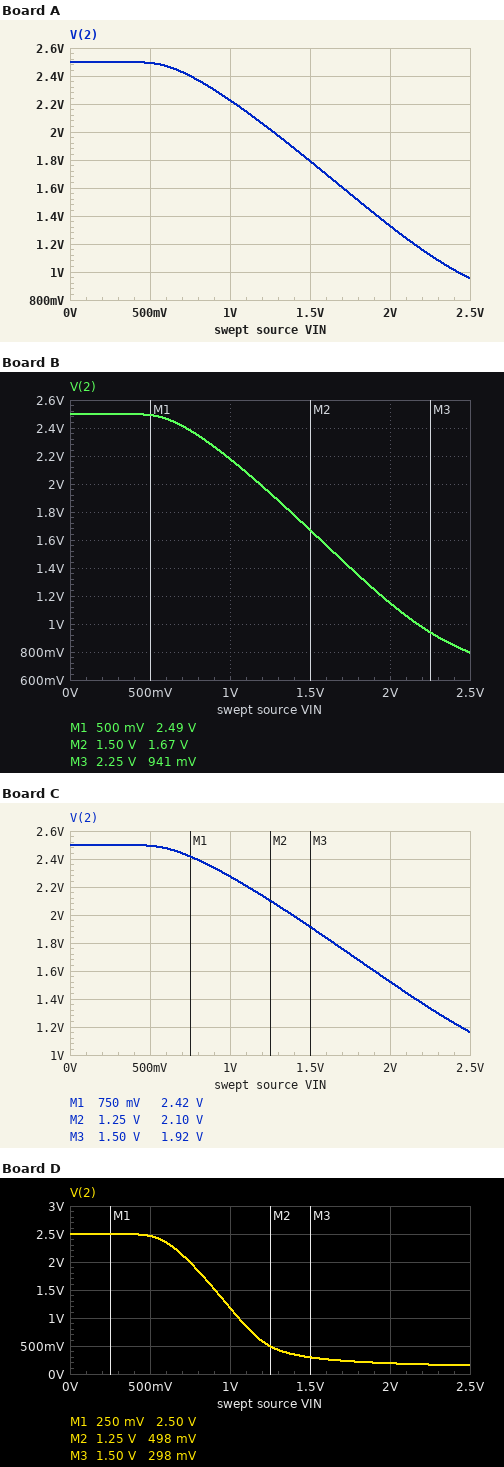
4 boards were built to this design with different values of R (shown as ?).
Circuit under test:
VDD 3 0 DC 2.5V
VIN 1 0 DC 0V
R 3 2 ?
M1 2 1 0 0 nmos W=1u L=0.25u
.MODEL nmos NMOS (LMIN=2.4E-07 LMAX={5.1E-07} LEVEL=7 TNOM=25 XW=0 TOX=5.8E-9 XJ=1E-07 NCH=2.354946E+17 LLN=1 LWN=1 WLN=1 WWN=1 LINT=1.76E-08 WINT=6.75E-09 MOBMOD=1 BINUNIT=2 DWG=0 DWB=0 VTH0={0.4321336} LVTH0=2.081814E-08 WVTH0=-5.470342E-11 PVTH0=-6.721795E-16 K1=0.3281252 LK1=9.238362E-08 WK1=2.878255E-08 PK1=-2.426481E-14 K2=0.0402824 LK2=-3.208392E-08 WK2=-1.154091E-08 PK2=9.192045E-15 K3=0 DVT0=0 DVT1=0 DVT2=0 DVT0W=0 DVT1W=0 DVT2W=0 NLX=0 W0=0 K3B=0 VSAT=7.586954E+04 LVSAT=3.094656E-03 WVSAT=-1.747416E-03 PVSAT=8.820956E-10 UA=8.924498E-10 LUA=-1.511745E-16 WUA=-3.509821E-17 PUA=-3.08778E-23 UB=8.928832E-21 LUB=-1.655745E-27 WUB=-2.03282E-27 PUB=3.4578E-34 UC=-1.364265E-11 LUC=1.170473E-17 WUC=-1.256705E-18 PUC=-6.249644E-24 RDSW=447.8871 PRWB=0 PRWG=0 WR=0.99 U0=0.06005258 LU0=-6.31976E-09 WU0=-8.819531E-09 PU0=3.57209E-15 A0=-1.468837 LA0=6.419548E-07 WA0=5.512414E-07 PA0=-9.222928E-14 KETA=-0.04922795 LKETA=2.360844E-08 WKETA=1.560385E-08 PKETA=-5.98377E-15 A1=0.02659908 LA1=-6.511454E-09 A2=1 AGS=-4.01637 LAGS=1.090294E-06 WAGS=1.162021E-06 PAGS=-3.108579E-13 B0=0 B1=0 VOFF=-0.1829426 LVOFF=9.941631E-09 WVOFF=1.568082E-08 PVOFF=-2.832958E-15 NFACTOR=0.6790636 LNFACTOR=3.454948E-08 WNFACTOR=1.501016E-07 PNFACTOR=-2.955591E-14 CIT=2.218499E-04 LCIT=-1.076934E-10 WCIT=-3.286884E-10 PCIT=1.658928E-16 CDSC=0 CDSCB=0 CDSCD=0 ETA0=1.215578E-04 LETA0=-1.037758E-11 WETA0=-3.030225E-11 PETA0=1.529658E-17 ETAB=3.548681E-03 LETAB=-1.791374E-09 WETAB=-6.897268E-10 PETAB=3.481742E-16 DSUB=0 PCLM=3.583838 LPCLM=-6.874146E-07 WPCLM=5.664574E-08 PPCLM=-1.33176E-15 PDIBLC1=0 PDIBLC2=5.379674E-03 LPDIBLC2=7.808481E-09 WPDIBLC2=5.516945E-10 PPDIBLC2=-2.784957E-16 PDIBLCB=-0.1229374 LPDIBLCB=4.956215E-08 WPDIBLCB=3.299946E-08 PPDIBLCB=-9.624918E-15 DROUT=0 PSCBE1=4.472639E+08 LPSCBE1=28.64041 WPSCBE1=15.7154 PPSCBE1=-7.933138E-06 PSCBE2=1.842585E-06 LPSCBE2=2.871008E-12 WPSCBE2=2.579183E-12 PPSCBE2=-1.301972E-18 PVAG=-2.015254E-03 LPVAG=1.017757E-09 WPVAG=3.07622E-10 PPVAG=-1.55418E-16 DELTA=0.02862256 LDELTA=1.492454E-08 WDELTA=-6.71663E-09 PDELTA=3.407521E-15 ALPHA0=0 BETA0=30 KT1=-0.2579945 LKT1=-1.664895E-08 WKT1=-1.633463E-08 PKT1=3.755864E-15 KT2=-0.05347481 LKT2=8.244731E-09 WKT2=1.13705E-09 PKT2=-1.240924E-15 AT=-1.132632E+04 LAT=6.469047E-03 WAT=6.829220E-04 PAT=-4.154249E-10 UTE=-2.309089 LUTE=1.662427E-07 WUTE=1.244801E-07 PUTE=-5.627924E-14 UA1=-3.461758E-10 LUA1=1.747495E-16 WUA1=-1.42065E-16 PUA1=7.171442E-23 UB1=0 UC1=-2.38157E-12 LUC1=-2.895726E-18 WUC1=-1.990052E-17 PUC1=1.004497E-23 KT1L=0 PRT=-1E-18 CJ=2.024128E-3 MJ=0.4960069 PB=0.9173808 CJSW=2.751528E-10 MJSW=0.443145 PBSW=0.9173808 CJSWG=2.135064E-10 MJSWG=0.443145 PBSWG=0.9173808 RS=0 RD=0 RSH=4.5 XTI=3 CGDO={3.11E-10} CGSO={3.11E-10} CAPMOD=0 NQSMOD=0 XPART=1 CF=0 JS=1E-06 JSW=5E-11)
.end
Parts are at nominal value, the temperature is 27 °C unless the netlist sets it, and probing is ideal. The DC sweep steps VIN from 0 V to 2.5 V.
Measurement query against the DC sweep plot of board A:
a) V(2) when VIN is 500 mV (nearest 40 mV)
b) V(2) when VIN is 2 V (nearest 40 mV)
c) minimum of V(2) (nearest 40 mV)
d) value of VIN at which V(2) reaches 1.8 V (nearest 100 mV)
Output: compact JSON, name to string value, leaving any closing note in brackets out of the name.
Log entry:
{"V(2) when VIN is 500 mV": "2.48 V", "V(2) when VIN is 2 V": "1.32 V", "minimum of V(2)": "960 mV", "value of VIN at which V(2) reaches 1.8 V": "1.5 V"}
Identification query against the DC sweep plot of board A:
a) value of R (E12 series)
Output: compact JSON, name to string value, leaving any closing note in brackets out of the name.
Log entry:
{"value of R": "3.3 kΩ"}
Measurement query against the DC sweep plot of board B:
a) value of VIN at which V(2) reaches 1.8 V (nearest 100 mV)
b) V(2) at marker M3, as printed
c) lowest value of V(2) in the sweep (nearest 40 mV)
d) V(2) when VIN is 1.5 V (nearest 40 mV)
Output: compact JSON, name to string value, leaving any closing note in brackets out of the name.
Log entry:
{"value of VIN at which V(2) reaches 1.8 V": "1.4 V", "V(2) at marker M3, as printed": "941 mV", "lowest value of V(2) in the sweep": "800 mV", "V(2) when VIN is 1.5 V": "1.68 V"}
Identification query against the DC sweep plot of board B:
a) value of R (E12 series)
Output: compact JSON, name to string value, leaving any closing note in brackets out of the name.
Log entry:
{"value of R": "3.9 kΩ"}
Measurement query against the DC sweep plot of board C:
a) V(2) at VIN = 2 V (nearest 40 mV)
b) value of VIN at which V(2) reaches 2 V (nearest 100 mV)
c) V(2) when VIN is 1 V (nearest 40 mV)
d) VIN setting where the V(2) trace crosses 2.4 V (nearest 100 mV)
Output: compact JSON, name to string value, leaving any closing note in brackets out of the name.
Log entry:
{"V(2) at VIN = 2 V": "1.52 V", "value of VIN at which V(2) reaches 2 V": "1.4 V", "V(2) when VIN is 1 V": "2.28 V", "VIN setting where the V(2) trace crosses 2.4 V": "800 mV"}
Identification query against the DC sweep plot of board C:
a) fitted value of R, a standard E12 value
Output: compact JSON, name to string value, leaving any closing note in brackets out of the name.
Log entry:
{"fitted value of R, a standard E12 value": "2.7 kΩ"}
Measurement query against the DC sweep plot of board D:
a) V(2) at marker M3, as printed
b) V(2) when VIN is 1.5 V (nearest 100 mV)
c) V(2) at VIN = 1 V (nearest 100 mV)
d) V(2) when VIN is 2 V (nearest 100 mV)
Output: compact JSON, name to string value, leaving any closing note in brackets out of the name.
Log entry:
{"V(2) at marker M3, as printed": "298 mV", "V(2) when VIN is 1.5 V": "300 mV", "V(2) at VIN = 1 V": "1.2 V", "V(2) when VIN is 2 V": "200 mV"}
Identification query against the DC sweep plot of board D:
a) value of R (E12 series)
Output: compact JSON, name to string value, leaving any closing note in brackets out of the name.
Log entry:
{"value of R": "18 kΩ"}
